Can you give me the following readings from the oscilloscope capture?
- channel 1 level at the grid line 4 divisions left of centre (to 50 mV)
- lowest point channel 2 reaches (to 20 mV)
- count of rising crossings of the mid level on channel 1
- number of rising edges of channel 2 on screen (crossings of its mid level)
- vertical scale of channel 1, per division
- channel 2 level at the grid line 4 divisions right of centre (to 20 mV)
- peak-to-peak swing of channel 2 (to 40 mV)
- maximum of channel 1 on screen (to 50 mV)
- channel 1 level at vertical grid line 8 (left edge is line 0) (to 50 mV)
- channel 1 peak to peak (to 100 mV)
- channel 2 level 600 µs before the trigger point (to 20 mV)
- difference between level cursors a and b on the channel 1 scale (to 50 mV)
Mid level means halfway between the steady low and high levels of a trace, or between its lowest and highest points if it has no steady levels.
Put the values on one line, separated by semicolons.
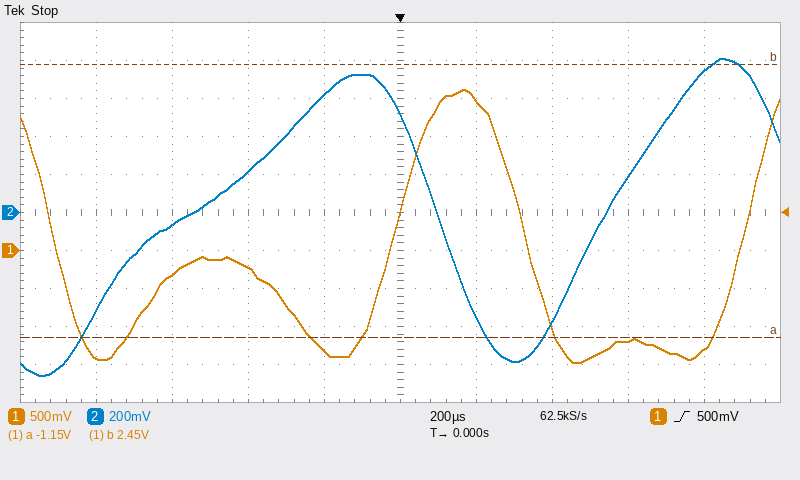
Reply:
-1.40 V; -860 mV; 2; 2; 500 mV; 740 mV; 1.68 V; 2.10 V; -1.20 V; 3.60 V; -60 mV; 3.60 V
